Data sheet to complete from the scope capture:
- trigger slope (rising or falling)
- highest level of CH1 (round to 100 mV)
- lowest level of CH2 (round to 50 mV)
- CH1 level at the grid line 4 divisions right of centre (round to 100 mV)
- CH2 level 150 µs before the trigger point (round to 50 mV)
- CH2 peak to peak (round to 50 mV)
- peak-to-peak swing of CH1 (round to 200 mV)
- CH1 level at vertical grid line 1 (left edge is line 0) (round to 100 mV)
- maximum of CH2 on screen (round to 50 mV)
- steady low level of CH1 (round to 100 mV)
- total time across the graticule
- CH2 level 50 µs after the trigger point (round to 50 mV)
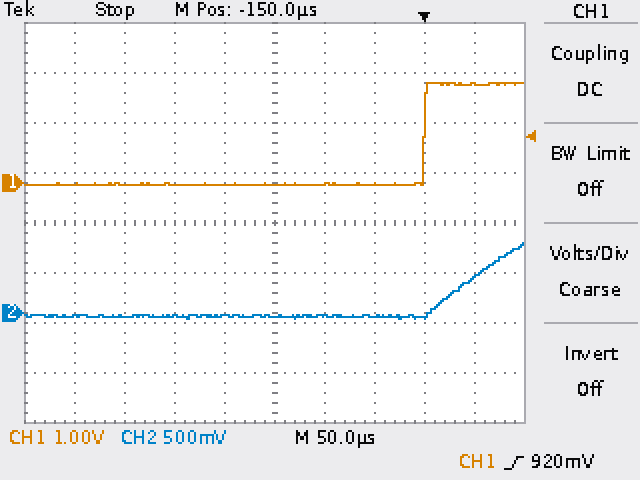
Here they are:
rising
2.0 V
-50 mV
2.0 V
-50 mV
750 mV
2.0 V
0.0 V
700 mV
0.0 V
500 µs
350 mV
